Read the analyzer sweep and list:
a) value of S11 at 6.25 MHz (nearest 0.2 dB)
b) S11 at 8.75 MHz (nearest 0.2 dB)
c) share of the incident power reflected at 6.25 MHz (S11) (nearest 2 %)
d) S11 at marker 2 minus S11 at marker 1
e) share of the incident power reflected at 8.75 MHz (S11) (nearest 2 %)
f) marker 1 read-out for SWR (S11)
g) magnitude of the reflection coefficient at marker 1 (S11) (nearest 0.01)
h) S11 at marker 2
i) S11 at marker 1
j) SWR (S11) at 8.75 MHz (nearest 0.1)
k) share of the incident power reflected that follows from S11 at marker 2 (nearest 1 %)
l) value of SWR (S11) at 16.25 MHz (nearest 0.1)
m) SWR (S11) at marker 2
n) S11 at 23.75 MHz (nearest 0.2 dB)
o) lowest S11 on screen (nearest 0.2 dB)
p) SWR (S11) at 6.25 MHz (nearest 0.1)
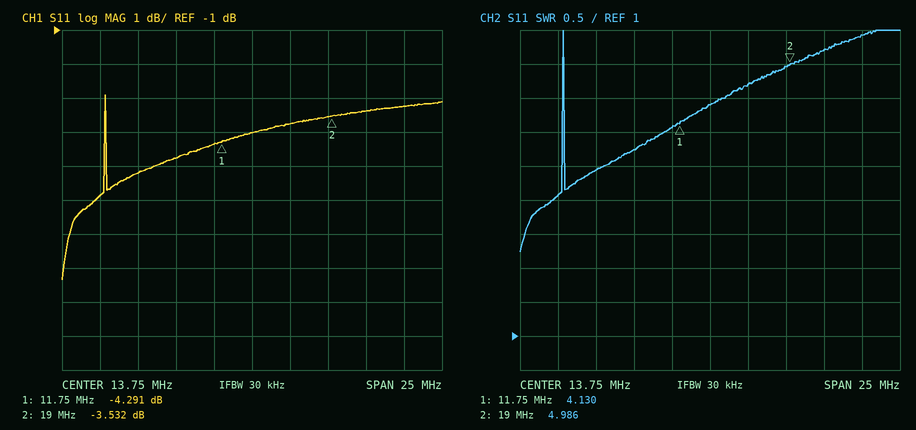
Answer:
-5.2 dB
-4.8 dB
30 %
0.759 dB
34 %
4.130
0.61
-3.532 dB
-4.291 dB
3.7
44 %
4.7
4.986
-3.2 dB
-8.4 dB
3.4
